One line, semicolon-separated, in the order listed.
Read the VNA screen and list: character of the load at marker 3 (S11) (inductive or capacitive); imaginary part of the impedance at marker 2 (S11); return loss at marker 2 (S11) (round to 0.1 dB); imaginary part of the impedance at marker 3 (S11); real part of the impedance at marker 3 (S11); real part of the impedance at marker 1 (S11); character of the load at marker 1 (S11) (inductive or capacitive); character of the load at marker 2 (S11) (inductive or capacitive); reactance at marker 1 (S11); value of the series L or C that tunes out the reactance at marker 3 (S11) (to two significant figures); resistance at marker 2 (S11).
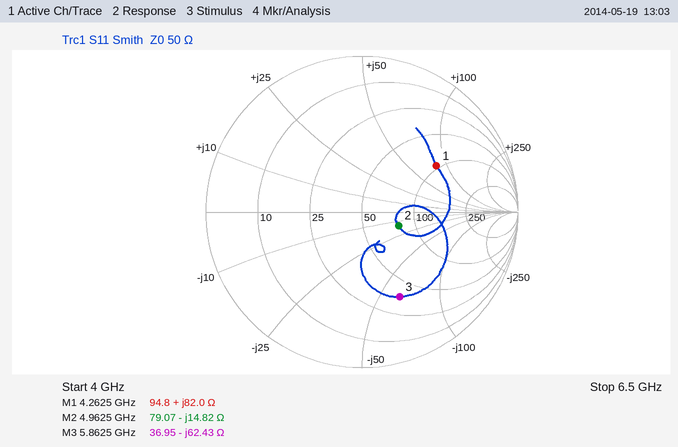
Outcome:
capacitive; -14.82 Ω; 12.0 dB; -62.43 Ω; 36.95 Ω; 94.8 Ω; inductive; capacitive; +82.0 Ω; 1.7 nH; 79.07 Ω
